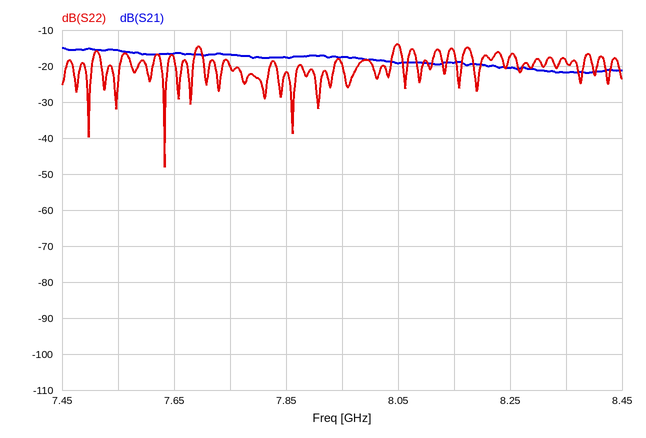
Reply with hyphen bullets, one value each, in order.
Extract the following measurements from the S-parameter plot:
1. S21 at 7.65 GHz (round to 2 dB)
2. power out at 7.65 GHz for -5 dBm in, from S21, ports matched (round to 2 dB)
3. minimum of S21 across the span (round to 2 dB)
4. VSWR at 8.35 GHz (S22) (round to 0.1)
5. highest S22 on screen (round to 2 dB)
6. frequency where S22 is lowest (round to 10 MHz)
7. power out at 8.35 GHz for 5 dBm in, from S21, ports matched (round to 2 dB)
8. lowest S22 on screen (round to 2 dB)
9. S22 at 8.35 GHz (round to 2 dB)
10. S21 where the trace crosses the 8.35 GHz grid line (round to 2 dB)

- -16 dB
- -22 dBm
- -22 dB
- 1.3
- -14 dB
- 7.63 GHz
- -16 dBm
- -48 dB
- -18 dB
- -22 dB
